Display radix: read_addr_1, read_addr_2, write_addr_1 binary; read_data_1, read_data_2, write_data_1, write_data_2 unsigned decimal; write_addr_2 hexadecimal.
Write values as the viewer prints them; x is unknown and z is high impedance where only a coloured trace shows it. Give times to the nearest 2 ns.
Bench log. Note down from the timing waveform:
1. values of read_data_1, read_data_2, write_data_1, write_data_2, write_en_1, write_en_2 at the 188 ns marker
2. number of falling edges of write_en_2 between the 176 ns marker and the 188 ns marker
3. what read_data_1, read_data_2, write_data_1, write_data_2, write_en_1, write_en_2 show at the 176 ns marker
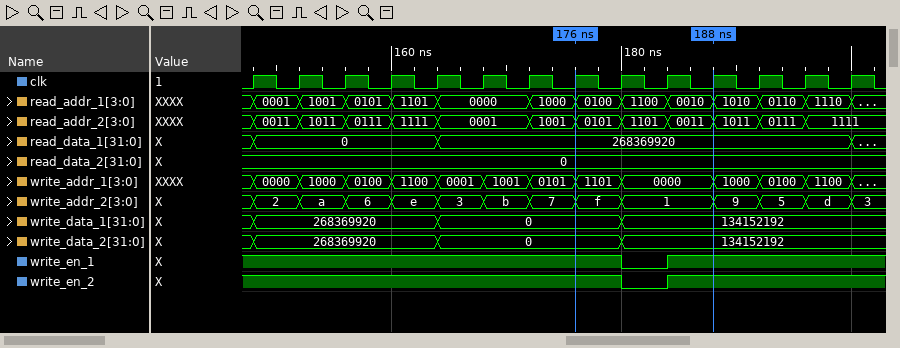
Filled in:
read_data_1=268369920, read_data_2=0, write_data_1=134152192, write_data_2=134152192, write_en_1=1, write_en_2=1
1
read_data_1=268369920, read_data_2=0, write_data_1=0, write_data_2=0, write_en_1=1, write_en_2=1
